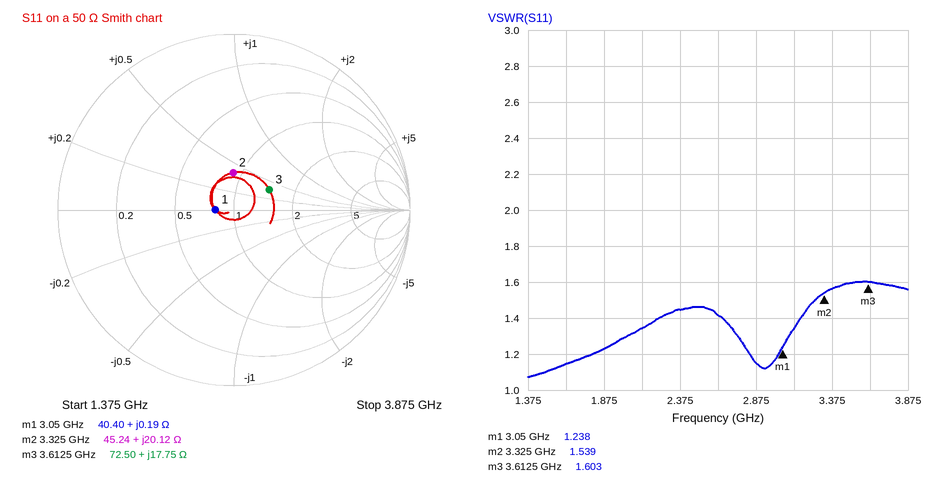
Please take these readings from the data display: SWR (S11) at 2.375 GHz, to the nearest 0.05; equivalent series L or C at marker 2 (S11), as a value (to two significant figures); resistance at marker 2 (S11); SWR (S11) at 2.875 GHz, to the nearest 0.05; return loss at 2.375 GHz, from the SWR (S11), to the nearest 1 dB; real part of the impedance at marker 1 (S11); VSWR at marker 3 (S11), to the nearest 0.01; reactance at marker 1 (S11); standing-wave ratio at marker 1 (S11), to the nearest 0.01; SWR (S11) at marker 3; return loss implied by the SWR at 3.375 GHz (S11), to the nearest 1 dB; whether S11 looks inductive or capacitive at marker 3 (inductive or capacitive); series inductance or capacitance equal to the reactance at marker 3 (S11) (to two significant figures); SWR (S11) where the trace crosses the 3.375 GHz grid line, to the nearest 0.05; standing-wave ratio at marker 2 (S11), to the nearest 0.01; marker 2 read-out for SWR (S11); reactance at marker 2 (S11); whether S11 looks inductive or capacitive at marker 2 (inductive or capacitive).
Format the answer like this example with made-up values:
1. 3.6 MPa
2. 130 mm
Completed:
1. 1.45
2. 960 pH
3. 45.24 Ω
4. 1.15
5. 15 dB
6. 40.40 Ω
7. 1.60
8. +0.19 Ω
9. 1.24
10. 1.603
11. 13 dB
12. inductive
13. 780 pH
14. 1.55
15. 1.54
16. 1.539
17. +20.12 Ω
18. inductive
